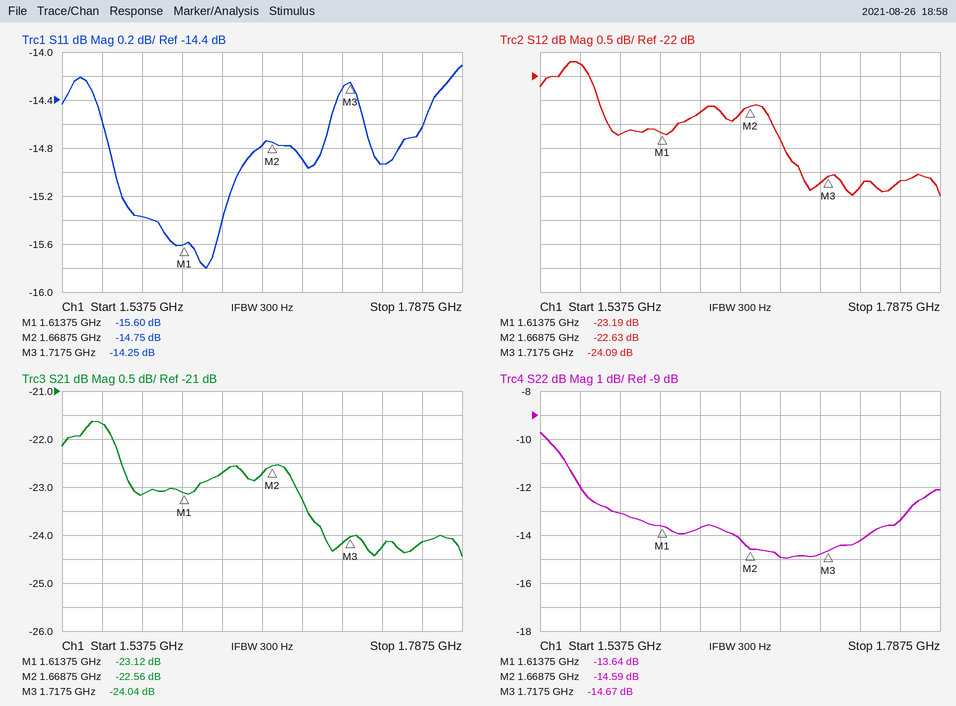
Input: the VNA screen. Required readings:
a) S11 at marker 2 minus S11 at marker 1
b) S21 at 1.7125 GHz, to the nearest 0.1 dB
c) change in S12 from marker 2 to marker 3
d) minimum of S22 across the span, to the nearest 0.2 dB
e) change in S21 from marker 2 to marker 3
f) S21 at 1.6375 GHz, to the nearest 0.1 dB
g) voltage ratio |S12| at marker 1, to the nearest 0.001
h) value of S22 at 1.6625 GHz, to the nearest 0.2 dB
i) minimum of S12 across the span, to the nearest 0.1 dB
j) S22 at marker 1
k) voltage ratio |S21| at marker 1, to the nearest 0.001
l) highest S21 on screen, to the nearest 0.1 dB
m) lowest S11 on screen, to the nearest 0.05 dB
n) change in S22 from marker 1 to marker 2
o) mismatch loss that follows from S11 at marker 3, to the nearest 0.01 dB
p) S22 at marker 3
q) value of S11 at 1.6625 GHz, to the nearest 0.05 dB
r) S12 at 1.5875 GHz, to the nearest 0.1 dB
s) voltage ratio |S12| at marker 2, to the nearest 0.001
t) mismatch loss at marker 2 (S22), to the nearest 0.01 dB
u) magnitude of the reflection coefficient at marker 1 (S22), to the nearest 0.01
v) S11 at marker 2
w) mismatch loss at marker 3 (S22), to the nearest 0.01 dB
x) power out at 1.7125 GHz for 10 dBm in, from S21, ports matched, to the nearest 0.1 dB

0.85 dB
-24.2 dB
-1.46 dB
-15.0 dB
-1.48 dB
-22.7 dB
0.069
-14.2 dB
-24.5 dB
-13.64 dB
0.070
-21.6 dB
-15.80 dB
-0.95 dB
0.17 dB
-14.67 dB
-14.80 dB
-23.2 dB
0.074
0.15 dB
0.21
-14.75 dB
0.15 dB
-14.2 dBm
